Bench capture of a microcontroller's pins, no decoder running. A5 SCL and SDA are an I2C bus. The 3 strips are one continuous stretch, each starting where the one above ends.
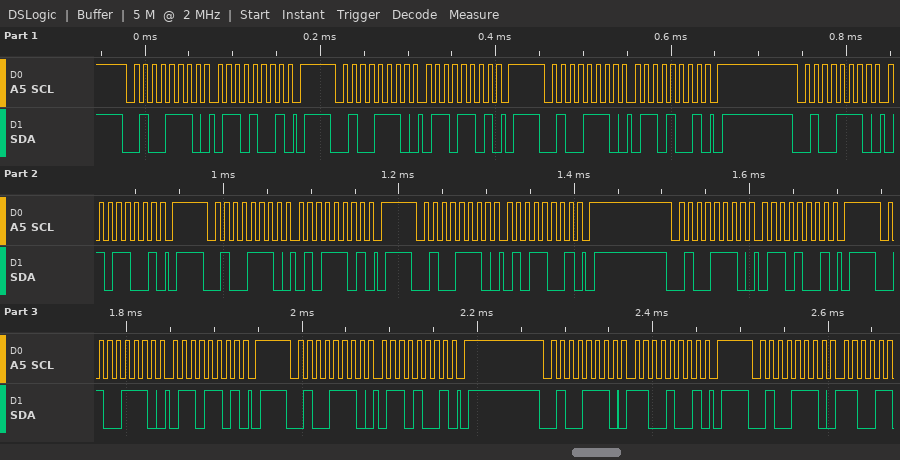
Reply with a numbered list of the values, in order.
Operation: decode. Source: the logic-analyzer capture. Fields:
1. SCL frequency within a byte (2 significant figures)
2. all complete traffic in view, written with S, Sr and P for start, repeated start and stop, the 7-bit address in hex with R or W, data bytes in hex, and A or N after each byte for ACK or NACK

1. 100 kHz
2. S 27W A 69 A P S 27W A 6D A P S 27W A 69 A P S 27W A 59 A P S 27W A 5D A P S 27W A 59 A P S 27W A 69 A P S 27W A 6D A P S 27W A 69 A P S 27W A C9 A P S 27W A
